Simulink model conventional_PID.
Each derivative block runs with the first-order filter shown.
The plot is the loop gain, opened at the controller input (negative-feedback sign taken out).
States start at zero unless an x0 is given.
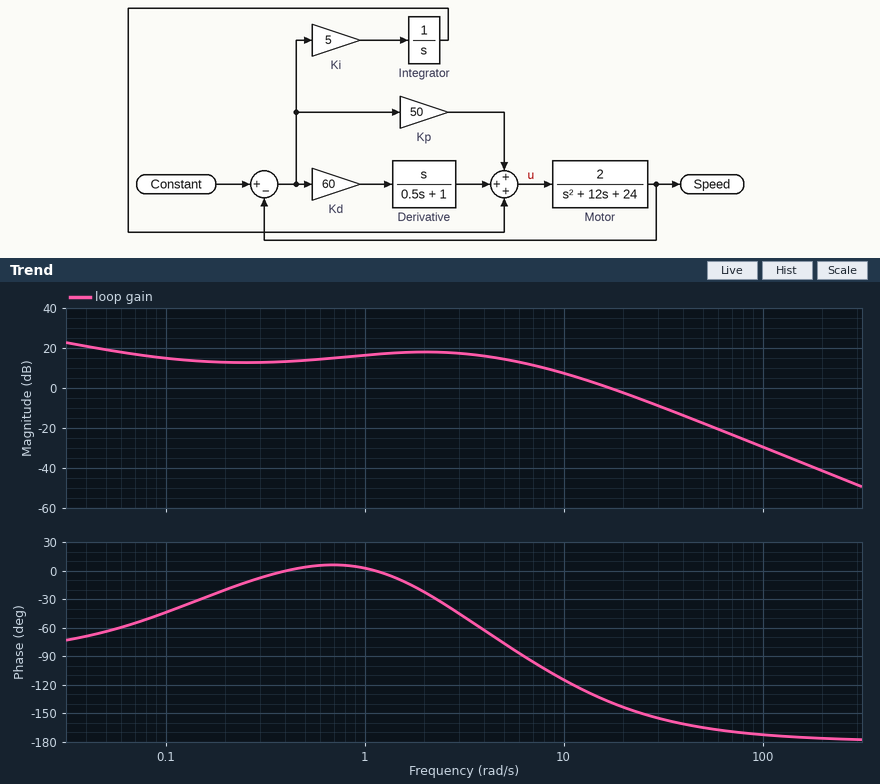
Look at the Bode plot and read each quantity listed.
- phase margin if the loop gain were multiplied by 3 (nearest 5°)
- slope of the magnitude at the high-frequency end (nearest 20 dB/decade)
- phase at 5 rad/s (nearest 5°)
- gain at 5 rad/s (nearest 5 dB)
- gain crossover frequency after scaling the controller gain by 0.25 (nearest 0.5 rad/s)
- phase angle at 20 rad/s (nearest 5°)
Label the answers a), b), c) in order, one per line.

a) 25°
b) -40 dB/decade
c) -75°
d) 15 dB
e) 6.5 rad/s
f) -145°
